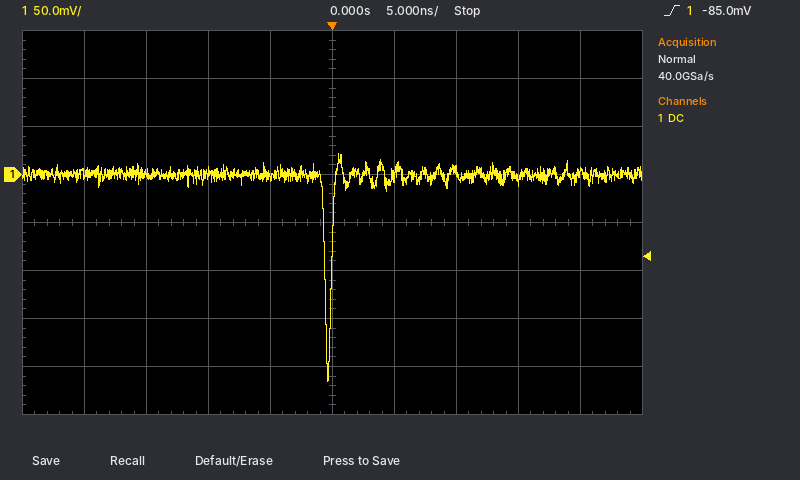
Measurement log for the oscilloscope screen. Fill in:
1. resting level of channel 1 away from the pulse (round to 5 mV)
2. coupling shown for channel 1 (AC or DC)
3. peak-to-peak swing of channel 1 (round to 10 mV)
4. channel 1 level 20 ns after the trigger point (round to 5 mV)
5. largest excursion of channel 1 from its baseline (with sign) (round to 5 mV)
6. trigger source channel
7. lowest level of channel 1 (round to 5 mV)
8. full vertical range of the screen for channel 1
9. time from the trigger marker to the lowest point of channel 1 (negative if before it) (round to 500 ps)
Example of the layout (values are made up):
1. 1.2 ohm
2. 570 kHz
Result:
1. 0 mV
2. DC
3. 240 mV
4. 0 mV
5. -215 mV
6. channel 1
7. -215 mV
8. 400 mV
9. -500 ps
